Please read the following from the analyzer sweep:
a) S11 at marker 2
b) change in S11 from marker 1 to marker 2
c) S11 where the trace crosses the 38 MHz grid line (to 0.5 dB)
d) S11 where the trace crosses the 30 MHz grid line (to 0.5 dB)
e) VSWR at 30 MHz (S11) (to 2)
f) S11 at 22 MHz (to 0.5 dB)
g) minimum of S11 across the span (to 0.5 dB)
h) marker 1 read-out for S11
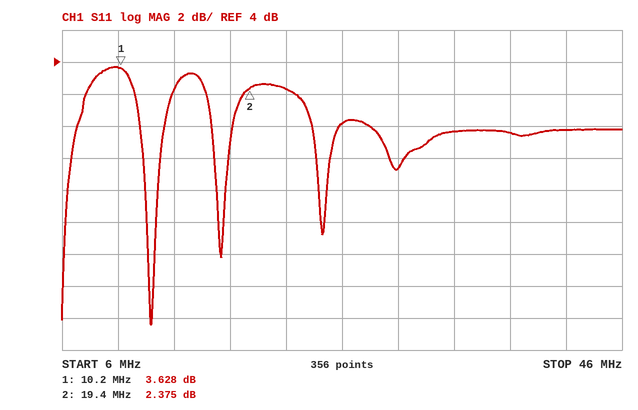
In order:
2.375 dB
-1.253 dB
-0.5 dB
-2.5 dB
6
2.5 dB
-12.5 dB
3.628 dB
